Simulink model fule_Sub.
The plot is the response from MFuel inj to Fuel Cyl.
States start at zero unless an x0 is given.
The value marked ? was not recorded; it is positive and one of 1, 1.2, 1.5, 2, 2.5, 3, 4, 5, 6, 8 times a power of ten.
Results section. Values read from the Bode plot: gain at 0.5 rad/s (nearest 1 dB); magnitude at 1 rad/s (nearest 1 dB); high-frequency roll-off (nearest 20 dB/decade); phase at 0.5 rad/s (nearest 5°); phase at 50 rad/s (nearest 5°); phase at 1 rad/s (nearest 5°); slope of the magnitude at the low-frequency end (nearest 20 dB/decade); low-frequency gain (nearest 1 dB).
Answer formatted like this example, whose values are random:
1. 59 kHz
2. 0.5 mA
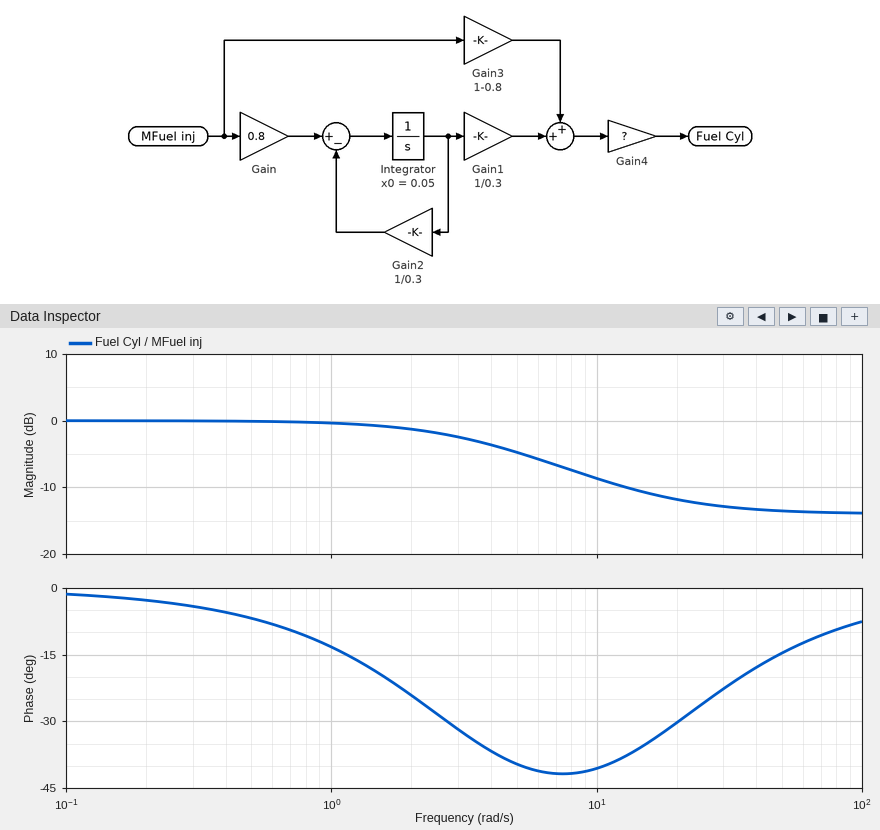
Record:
1. 0 dB
2. 0 dB
3. 0 dB/decade
4. -5°
5. -15°
6. -15°
7. 0 dB/decade
8. 0 dB
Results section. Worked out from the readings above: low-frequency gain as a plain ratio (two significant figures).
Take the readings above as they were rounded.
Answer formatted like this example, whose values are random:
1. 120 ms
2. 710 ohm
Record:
1. 1.0
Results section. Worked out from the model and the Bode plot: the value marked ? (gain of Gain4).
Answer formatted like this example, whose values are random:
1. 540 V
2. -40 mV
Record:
1. 1
